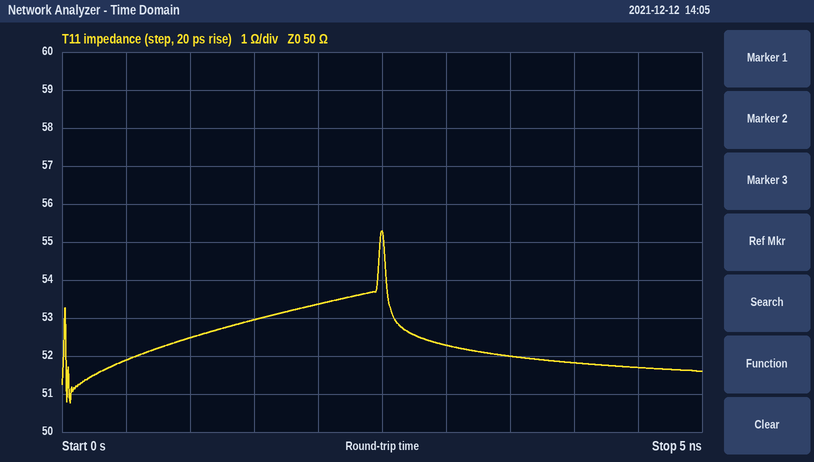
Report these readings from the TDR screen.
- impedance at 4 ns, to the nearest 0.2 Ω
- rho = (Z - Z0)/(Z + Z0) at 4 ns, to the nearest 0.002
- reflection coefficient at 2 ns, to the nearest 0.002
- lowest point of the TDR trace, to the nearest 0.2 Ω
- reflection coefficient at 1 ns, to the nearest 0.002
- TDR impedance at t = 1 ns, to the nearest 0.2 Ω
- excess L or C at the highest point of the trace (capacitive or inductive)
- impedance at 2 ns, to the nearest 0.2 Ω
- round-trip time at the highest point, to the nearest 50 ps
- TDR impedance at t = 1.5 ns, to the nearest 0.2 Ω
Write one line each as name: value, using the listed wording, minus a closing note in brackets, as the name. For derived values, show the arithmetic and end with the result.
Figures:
impedance at 4 ns, to the nearest 0.2 Ω: 51.8 Ω
rho = (Z - Z0)/(Z + Z0) at 4 ns, to the nearest 0.002: (51.8 − 50)/(51.8 + 50) ≈ +0.018
reflection coefficient at 2 ns, to the nearest 0.002: (53.4 − 50)/(53.4 + 50) ≈ +0.0329, so +0.032 to the nearest 0.002
lowest point of the TDR trace, to the nearest 0.2 Ω: 50.8 Ω
reflection coefficient at 1 ns, to the nearest 0.002: (52.4 − 50)/(52.4 + 50) ≈ +0.0234, so +0.024 to the nearest 0.002
TDR impedance at t = 1 ns, to the nearest 0.2 Ω: 52.4 Ω
excess L or C at the highest point of the trace: inductive
impedance at 2 ns, to the nearest 0.2 Ω: 53.4 Ω
round-trip time at the highest point, to the nearest 50 ps: 2.50 ns
TDR impedance at t = 1.5 ns, to the nearest 0.2 Ω: 53.0 Ω
